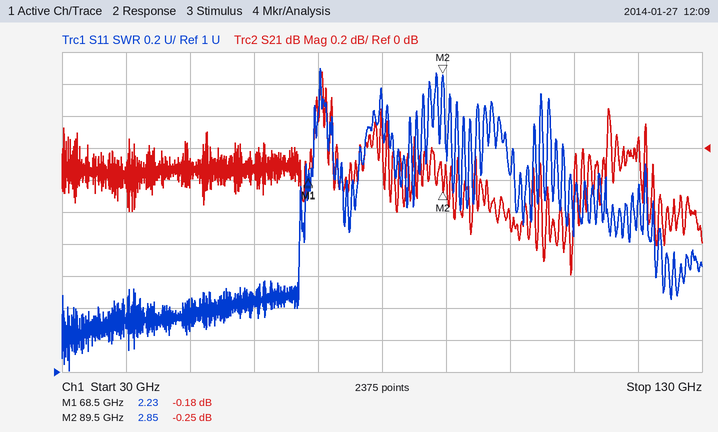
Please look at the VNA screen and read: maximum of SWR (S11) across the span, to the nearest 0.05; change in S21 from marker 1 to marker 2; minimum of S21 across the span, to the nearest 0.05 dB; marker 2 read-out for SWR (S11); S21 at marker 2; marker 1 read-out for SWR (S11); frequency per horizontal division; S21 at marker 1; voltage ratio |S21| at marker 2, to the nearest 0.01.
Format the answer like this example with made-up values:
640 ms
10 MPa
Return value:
2.90
-0.07 dB
-0.80 dB
2.85
-0.25 dB
2.23
10 GHz
-0.18 dB
0.97
